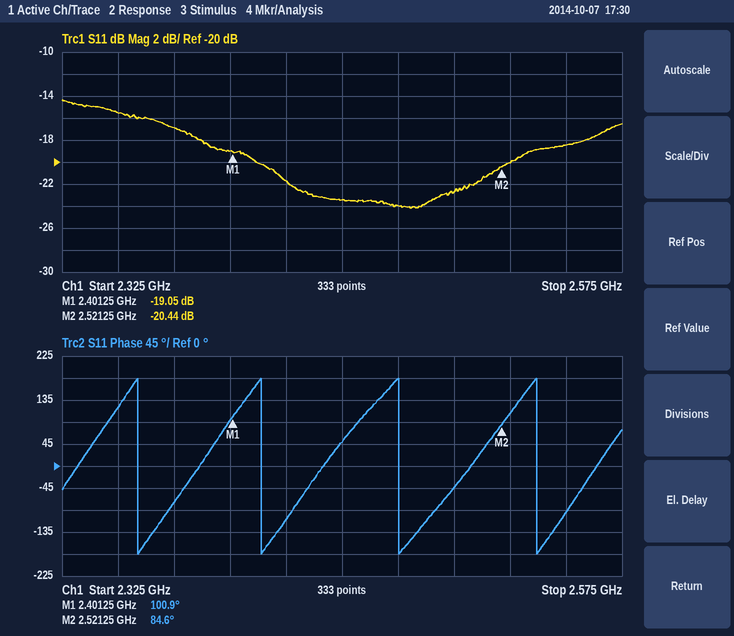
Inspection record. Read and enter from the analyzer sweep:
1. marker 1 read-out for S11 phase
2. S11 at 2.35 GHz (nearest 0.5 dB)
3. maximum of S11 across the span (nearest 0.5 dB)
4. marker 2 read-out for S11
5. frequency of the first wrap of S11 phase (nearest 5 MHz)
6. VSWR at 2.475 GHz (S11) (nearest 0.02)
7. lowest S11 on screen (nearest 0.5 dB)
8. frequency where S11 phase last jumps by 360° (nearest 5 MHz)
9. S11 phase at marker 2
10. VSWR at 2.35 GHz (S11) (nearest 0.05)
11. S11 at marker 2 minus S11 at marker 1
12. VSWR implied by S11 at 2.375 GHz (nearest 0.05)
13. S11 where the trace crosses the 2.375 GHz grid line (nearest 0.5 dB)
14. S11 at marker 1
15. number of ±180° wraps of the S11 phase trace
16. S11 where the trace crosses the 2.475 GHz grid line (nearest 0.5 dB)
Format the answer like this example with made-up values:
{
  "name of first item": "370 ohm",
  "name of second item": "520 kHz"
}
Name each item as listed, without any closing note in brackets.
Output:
{
  "marker 1 read-out for S11 phase": "100.9°",
  "S11 at 2.35 GHz": "-15.5 dB",
  "maximum of S11 across the span": "-14.5 dB",
  "marker 2 read-out for S11": "-20.44 dB",
  "frequency of the first wrap of S11 phase": "2.360 GHz",
  "VSWR at 2.475 GHz (S11)": "1.14",
  "lowest S11 on screen": "-24.0 dB",
  "frequency where S11 phase last jumps by 360°": "2.535 GHz",
  "S11 phase at marker 2": "84.6°",
  "VSWR at 2.35 GHz (S11)": "1.40",
  "S11 at marker 2 minus S11 at marker 1": "-1.39 dB",
  "VSWR implied by S11 at 2.375 GHz": "1.35",
  "S11 where the trace crosses the 2.375 GHz grid line": "-17.0 dB",
  "S11 at marker 1": "-19.05 dB",
  "number of ±180° wraps of the S11 phase trace": "4",
  "S11 where the trace crosses the 2.475 GHz grid line": "-24.0 dB"
}
